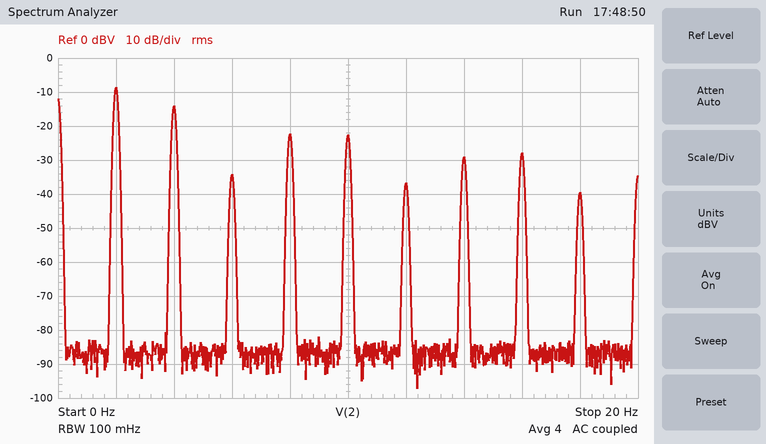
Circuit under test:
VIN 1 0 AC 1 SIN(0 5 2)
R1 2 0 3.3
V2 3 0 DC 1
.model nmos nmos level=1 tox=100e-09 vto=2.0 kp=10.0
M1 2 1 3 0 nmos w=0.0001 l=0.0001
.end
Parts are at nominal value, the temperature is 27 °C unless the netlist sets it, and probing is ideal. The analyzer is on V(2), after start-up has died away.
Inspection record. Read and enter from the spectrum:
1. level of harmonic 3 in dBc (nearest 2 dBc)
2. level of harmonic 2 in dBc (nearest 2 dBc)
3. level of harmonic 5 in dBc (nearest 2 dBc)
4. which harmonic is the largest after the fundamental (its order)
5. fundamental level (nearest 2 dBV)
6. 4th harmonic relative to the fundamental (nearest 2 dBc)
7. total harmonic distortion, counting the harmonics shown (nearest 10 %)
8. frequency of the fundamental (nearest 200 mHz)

-26 dBc
-6 dBc
-14 dBc
2
-8 dBV
-14 dBc
60 %
2.0 Hz
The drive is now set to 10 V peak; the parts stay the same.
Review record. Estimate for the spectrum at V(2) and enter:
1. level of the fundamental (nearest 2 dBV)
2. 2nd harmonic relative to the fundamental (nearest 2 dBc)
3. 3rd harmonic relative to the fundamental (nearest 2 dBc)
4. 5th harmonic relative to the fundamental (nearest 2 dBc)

-8 dBV
-12 dBc
-12 dBc
-28 dBc
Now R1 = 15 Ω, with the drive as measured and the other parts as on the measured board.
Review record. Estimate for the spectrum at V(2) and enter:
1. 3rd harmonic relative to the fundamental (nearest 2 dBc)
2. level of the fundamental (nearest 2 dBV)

-32 dBc
-8 dBV
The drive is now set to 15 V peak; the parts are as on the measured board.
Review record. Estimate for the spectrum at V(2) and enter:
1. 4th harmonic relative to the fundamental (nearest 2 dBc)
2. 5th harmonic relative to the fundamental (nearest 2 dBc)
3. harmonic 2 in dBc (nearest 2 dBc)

-16 dBc
-18 dBc
-14 dBc
